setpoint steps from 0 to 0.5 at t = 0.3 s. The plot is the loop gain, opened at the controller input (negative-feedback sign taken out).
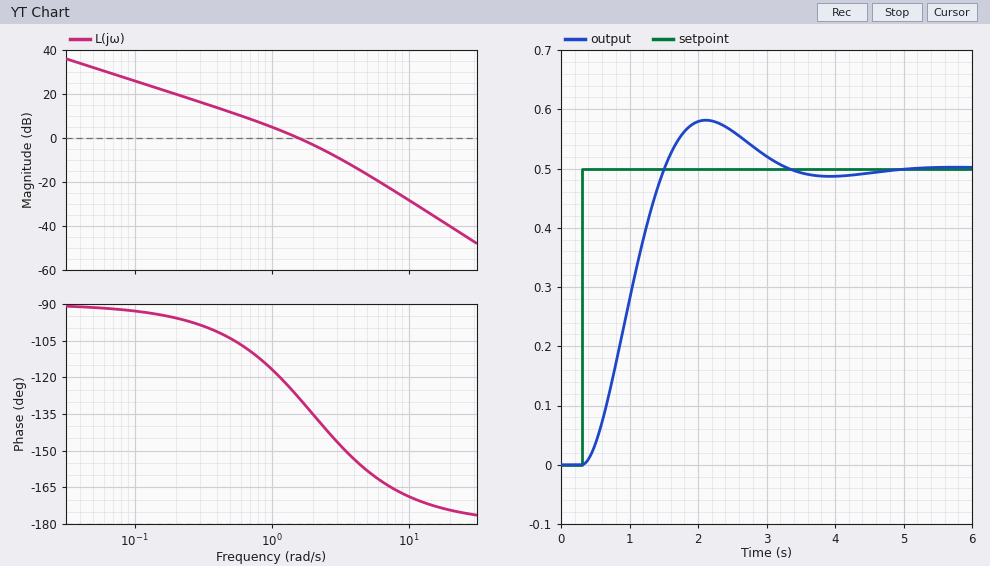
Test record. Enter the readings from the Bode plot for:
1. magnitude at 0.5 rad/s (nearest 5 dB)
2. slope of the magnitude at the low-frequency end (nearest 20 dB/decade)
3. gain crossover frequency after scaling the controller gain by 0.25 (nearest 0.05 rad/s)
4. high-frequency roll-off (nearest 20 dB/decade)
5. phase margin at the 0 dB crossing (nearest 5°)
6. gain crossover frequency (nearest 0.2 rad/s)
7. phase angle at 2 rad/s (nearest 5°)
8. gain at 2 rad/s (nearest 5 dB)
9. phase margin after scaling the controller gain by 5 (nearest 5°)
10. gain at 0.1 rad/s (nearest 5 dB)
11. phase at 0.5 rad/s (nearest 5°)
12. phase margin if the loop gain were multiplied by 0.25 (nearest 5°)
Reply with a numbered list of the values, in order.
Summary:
1. 10 dB
2. -20 dB/decade
3. 0.50 rad/s
4. -40 dB/decade
5. 50°
6. 1.6 rad/s
7. -135°
8. -5 dB
9. 25°
10. 25 dB
11. -105°
12. 75°
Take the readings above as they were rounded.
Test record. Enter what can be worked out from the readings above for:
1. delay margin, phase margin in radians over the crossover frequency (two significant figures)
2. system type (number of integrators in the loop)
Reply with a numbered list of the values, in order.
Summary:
1. 0.55 s
2. 1
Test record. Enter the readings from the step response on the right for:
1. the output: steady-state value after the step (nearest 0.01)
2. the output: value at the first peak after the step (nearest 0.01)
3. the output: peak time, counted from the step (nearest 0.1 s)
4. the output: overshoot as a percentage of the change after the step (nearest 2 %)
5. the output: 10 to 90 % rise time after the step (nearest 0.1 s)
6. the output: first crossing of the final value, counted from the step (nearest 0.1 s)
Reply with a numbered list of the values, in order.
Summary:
1. 0.50
2. 0.58
3. 1.8 s
4. 16 %
5. 0.8 s
6. 1.2 s
